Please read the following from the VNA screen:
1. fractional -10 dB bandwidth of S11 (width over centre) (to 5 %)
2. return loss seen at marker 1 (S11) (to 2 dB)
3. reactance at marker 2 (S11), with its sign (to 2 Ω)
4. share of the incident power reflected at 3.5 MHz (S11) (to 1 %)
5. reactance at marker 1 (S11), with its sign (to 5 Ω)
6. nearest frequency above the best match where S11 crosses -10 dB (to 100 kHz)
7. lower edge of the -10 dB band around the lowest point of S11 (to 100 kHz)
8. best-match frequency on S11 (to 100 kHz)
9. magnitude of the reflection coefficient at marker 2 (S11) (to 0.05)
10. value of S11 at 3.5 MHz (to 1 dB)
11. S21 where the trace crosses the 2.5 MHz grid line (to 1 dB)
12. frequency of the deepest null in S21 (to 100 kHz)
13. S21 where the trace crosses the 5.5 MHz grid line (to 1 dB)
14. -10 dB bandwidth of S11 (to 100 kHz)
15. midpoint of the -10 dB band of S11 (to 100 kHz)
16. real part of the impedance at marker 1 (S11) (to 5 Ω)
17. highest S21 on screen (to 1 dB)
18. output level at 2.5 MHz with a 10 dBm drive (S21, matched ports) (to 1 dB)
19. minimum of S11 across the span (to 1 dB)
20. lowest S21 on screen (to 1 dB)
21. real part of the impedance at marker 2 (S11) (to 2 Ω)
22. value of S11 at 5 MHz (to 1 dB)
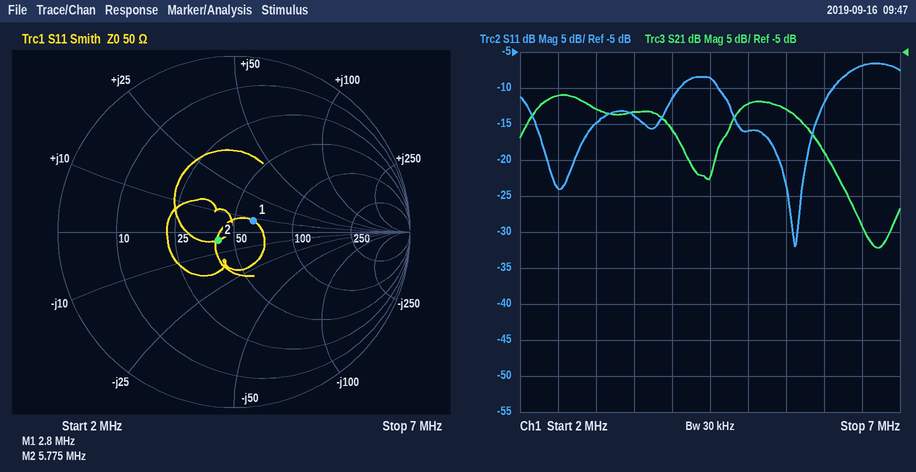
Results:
30 %
18 dB
-4 Ω
4 %
+10 Ω
6.1 MHz
4.6 MHz
5.6 MHz
0.10
-14 dB
-11 dB
6.7 MHz
-13 dB
1.5 MHz
5.4 MHz
60 Ω
-11 dB
-1 dBm
-32 dB
-32 dB
42 Ω
-16 dB
